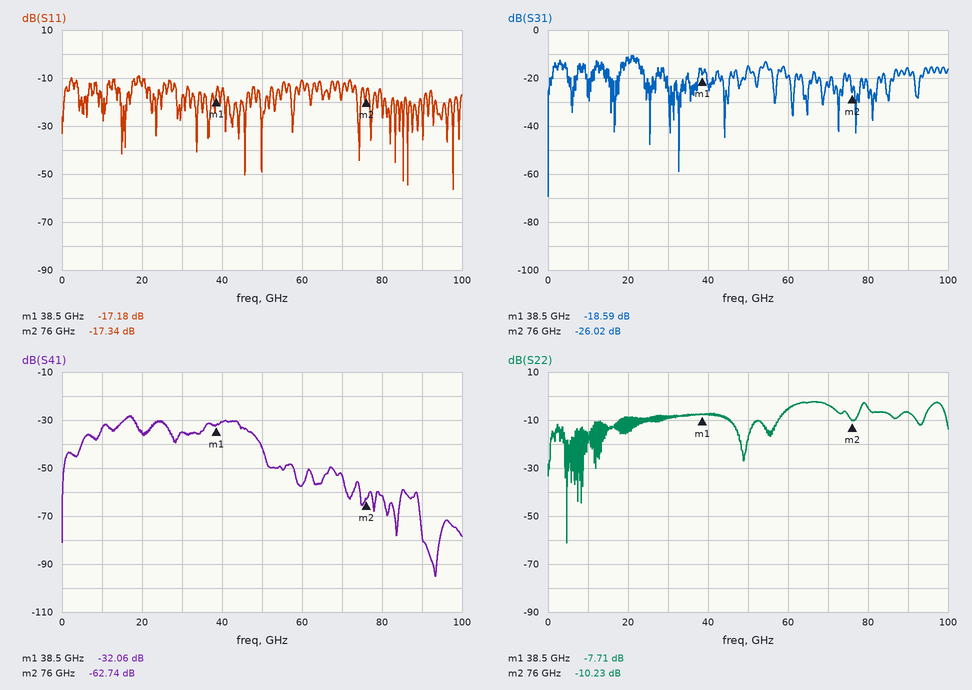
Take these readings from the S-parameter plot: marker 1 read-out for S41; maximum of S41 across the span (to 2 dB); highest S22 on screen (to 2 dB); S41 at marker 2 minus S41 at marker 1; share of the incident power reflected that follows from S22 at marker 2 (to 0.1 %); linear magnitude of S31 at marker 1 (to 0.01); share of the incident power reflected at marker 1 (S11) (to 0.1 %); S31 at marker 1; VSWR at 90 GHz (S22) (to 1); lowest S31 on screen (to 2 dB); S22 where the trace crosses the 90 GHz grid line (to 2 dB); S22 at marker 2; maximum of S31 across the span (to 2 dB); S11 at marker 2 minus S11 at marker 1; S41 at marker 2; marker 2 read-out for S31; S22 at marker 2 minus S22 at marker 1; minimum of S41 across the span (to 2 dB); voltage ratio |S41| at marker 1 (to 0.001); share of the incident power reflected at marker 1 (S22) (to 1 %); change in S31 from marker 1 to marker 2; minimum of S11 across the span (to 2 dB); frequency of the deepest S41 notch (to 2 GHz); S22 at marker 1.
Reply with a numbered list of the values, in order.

1. -32.06 dB
2. -28 dB
3. -2 dB
4. -30.68 dB
5. 9.5 %
6. 0.12
7. 1.9 %
8. -18.59 dB
9. 3
10. -70 dB
11. -6 dB
12. -10.23 dB
13. -10 dB
14. -0.16 dB
15. -62.74 dB
16. -26.02 dB
17. -2.52 dB
18. -96 dB
19. 0.025
20. 17 %
21. -7.43 dB
22. -56 dB
23. 94 GHz
24. -7.71 dB
